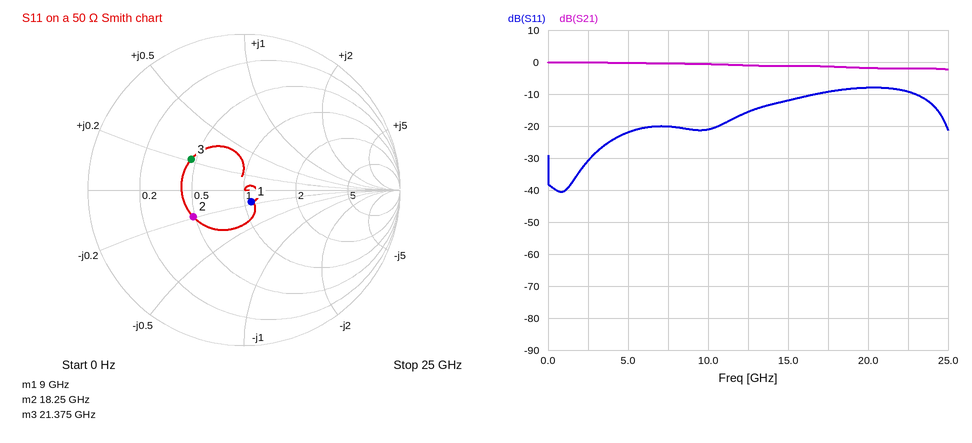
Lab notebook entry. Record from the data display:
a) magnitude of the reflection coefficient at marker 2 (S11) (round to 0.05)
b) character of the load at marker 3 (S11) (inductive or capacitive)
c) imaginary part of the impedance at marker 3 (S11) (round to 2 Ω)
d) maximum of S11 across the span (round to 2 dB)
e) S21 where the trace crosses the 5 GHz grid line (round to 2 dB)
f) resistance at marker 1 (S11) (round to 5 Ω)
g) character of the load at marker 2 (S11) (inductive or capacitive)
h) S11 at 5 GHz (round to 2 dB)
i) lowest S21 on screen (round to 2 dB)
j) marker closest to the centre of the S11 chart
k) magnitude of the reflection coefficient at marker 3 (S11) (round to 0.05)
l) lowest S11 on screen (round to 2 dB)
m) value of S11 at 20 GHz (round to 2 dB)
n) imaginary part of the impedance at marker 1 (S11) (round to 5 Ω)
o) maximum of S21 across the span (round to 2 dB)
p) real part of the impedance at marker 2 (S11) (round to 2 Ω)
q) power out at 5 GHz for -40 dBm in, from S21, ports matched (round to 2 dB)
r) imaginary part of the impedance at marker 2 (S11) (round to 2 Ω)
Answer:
0.35
inductive
+10 Ω
-8 dB
0 dB
55 Ω
capacitive
-22 dB
-2 dB
marker 1
0.40
-40 dB
-8 dB
-10 Ω
0 dB
24 Ω
-40 dBm
-10 Ω
